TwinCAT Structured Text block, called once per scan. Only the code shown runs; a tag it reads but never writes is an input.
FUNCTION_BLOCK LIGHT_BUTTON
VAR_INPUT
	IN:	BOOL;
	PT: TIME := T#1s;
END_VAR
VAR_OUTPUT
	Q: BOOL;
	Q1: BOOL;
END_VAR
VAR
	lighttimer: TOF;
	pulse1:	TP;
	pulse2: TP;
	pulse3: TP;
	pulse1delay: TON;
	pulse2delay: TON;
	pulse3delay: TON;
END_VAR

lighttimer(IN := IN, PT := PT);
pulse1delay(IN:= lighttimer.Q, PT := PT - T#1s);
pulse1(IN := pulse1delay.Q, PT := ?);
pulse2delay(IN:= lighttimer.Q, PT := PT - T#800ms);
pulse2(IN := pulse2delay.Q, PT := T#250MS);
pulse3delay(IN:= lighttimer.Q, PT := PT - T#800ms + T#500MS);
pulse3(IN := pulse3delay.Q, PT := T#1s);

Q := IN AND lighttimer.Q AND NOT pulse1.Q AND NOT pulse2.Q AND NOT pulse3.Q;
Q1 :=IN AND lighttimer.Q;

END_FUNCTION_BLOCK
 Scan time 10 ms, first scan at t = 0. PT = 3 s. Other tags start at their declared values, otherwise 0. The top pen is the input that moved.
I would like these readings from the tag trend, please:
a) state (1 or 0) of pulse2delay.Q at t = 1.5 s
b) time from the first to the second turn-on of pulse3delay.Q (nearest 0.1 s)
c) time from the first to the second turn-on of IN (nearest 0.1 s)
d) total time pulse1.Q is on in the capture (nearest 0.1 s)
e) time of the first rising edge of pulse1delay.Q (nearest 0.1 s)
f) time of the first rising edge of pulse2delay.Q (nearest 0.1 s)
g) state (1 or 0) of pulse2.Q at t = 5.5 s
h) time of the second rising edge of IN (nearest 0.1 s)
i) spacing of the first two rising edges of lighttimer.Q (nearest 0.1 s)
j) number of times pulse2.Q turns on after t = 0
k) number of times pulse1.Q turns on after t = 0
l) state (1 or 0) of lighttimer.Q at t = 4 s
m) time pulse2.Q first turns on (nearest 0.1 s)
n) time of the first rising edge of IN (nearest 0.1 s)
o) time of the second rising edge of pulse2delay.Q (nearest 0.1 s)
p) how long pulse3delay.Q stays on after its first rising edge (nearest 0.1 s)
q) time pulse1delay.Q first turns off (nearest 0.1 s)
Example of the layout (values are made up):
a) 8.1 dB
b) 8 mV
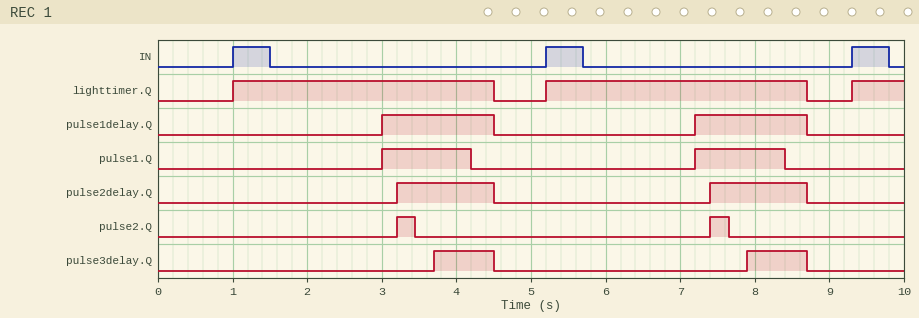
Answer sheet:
a) 0
b) 4.2 s
c) 4.2 s
d) 2.4 s
e) 3.0 s
f) 3.2 s
g) 0
h) 5.2 s
i) 4.2 s
j) 2
k) 2
l) 1
m) 3.2 s
n) 1.0 s
o) 7.4 s
p) 0.8 s
q) 4.5 s
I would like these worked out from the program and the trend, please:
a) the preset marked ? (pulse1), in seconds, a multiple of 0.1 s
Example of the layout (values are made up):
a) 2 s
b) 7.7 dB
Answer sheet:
a) 1.2 s
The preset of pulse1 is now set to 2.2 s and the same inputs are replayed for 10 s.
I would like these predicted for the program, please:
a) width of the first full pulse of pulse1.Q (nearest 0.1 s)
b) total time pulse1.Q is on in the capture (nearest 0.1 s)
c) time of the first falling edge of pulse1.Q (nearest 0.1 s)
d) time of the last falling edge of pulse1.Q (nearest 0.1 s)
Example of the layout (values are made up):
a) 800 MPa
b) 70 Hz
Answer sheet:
a) 2.2 s
b) 4.4 s
c) 5.2 s
d) 9.4 s
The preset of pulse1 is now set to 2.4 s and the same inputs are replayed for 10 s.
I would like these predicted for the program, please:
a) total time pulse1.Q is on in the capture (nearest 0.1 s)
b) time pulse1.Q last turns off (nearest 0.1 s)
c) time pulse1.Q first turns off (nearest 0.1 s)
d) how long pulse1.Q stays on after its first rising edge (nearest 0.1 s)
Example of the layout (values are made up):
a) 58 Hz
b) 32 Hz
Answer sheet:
a) 4.8 s
b) 9.6 s
c) 5.4 s
d) 2.4 s
